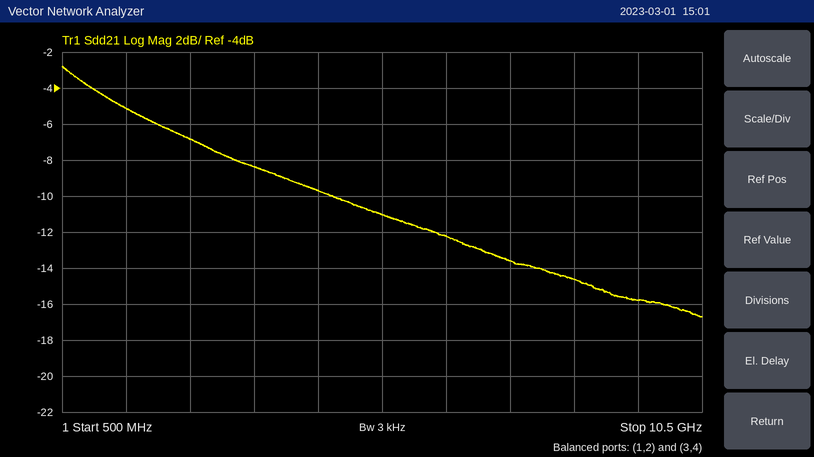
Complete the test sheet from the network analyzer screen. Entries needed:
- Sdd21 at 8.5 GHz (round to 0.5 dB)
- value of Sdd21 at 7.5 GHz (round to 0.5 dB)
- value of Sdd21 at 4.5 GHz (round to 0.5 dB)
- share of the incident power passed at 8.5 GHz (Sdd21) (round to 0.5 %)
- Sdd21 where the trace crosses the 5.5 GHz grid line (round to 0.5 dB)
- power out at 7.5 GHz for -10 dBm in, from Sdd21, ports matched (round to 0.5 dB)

-14.5 dB
-13.5 dB
-9.5 dB
3.5 %
-11.0 dB
-23.5 dBm
